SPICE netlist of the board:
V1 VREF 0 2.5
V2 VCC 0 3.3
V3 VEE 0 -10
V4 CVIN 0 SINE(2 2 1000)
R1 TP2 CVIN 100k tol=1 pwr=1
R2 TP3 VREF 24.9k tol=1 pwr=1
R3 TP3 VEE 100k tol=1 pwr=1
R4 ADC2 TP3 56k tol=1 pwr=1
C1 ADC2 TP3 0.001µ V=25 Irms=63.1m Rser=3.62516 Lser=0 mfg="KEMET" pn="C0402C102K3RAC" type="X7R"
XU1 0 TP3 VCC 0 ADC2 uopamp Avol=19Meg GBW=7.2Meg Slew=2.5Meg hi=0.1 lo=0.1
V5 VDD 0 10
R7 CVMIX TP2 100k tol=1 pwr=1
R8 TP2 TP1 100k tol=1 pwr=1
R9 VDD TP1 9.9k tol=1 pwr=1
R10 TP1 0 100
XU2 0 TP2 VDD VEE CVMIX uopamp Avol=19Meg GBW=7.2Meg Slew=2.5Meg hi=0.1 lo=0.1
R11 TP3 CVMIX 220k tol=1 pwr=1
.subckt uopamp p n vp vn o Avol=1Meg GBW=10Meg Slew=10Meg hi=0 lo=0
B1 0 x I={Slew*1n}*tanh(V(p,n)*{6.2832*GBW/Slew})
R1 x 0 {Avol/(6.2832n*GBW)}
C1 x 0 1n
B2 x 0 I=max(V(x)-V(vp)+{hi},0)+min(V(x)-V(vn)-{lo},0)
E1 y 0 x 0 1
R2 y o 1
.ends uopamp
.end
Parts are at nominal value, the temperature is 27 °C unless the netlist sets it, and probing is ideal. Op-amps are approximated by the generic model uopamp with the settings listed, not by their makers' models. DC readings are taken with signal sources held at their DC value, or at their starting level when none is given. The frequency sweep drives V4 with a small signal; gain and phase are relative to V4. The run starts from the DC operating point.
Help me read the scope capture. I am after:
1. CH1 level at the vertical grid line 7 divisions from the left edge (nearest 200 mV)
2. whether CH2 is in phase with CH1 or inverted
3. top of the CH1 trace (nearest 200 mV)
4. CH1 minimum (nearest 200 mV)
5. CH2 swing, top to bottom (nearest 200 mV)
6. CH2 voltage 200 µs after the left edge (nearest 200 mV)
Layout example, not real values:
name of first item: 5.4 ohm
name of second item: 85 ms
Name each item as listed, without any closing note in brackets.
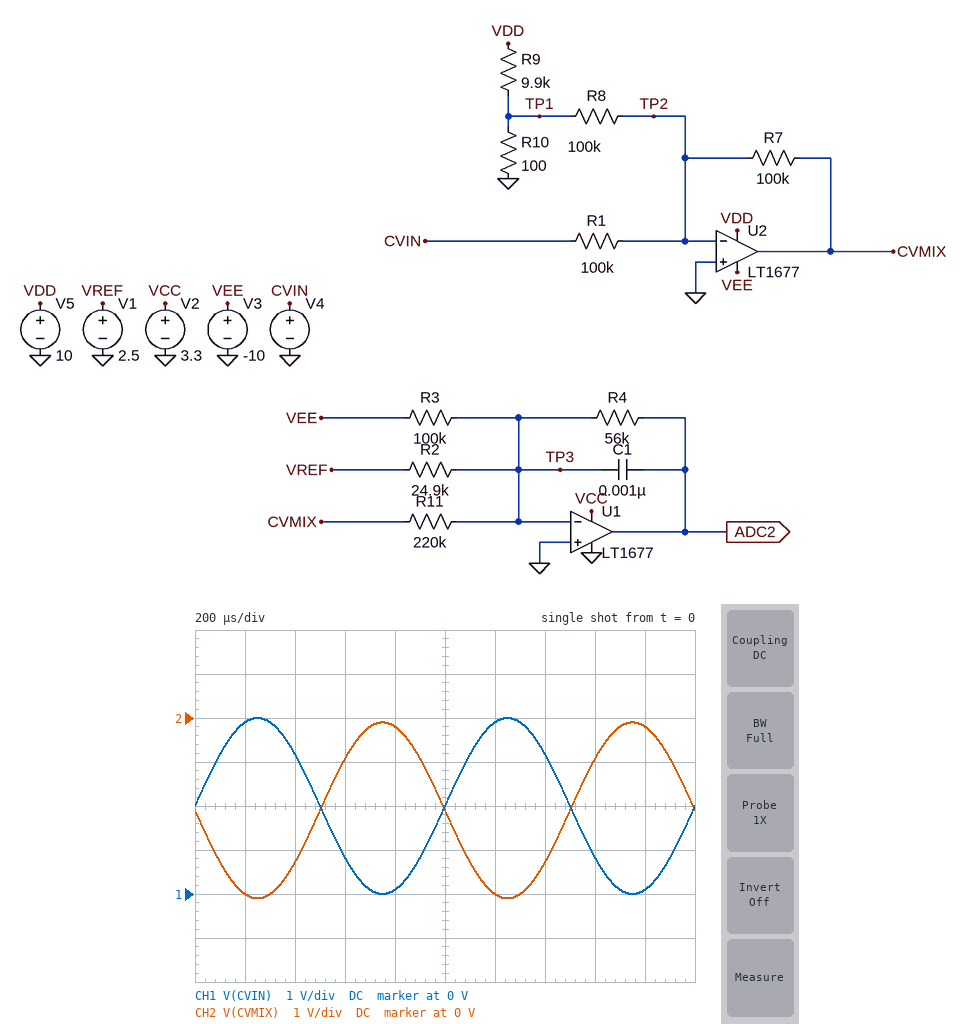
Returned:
CH1 level at the vertical grid line 7 divisions from the left edge: 3.2 V
whether CH2 is in phase with CH1 or inverted: inverted
top of the CH1 trace: 4.0 V
CH1 minimum: 0 V
CH2 swing, top to bottom: 4.0 V
CH2 voltage 200 µs after the left edge: -4.0 V
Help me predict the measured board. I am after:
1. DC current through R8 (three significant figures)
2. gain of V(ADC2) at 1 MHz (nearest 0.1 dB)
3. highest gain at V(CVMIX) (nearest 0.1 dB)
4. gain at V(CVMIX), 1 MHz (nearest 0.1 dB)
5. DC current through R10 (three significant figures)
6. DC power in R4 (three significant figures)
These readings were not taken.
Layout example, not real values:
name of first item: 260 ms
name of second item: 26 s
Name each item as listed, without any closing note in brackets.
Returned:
DC current through R8: 999 nA
gain of V(ADC2) at 1 MHz: -63.6 dB
highest gain at V(CVMIX): 0 dB
gain at V(CVMIX), 1 MHz: -0.7 dB
DC current through R10: 999 µA
DC power in R4: 4.68 µW
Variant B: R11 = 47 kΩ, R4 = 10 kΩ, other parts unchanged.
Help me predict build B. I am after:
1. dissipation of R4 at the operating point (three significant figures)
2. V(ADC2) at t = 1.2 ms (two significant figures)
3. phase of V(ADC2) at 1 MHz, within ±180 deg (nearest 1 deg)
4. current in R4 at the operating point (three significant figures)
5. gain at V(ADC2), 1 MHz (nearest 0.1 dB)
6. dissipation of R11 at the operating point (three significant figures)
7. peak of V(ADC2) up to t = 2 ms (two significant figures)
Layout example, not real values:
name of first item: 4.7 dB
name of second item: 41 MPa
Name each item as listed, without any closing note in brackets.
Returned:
dissipation of R4 at the operating point: 19.6 µW
V(ADC2) at t = 1.2 ms: 840 mV
phase of V(ADC2) at 1 MHz, within ±180 deg: -118 deg
current in R4 at the operating point: 44.3 µA
gain at V(ADC2), 1 MHz: -50.2 dB
dissipation of R11 at the operating point: 93.8 µW
peak of V(ADC2) up to t = 2 ms: 870 mV
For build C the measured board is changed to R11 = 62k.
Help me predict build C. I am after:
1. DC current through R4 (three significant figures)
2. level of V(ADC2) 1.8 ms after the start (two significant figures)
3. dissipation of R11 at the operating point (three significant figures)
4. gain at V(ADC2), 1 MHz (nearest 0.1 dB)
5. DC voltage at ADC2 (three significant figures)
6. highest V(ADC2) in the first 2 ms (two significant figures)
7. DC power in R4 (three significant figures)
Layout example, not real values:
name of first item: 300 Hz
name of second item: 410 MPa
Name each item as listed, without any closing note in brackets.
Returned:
DC current through R4: 33.5 µA
level of V(ADC2) 1.8 ms after the start: 170 mV
dissipation of R11 at the operating point: 71.1 µW
gain at V(ADC2), 1 MHz: -52.6 dB
DC voltage at ADC2: 1.87 V
highest V(ADC2) in the first 2 ms: 3.2 V
DC power in R4: 62.7 µW
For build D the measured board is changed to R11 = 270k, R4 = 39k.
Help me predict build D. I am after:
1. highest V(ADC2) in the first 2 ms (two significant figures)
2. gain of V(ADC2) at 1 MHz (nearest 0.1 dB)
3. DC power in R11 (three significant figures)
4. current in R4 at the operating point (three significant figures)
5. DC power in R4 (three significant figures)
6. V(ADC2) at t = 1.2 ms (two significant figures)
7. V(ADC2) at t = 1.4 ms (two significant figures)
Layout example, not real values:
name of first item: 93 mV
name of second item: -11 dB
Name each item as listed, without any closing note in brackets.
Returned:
highest V(ADC2) in the first 2 ms: 570 mV
gain of V(ADC2) at 1 MHz: -65.4 dB
DC power in R11: 16.3 µW
current in R4 at the operating point: 7.38 µA
DC power in R4: 2.12 µW
V(ADC2) at t = 1.2 ms: 530 mV
V(ADC2) at t = 1.4 ms: 500 mV
